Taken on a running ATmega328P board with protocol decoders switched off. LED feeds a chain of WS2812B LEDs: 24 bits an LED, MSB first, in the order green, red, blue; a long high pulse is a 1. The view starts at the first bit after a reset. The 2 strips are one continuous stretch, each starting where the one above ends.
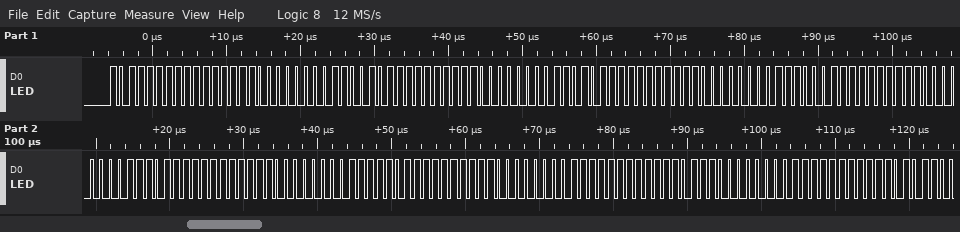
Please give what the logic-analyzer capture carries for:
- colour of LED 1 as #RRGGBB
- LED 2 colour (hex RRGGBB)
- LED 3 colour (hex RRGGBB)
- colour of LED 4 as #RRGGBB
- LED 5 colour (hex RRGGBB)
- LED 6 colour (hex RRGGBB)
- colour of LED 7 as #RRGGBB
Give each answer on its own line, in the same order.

#FFBF00
#FFCB00
#FFD700
#FFE300
#FFEF00
#FFFB00
#F7FF00
